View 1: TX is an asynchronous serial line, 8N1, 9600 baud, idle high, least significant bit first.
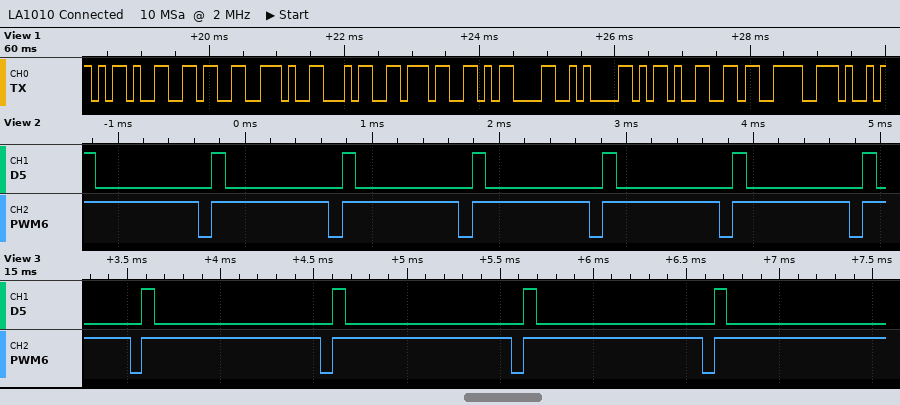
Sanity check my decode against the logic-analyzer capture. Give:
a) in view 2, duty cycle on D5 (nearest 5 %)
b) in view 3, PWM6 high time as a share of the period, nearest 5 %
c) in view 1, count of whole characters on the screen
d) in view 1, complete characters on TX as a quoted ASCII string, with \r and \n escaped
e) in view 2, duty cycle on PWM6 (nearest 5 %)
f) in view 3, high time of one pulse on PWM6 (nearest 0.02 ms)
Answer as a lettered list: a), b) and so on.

a) 10 %
b) 95 %
c) 10
d) "-6.47\r\n-6."
e) 90 %
f) 0.96 ms
